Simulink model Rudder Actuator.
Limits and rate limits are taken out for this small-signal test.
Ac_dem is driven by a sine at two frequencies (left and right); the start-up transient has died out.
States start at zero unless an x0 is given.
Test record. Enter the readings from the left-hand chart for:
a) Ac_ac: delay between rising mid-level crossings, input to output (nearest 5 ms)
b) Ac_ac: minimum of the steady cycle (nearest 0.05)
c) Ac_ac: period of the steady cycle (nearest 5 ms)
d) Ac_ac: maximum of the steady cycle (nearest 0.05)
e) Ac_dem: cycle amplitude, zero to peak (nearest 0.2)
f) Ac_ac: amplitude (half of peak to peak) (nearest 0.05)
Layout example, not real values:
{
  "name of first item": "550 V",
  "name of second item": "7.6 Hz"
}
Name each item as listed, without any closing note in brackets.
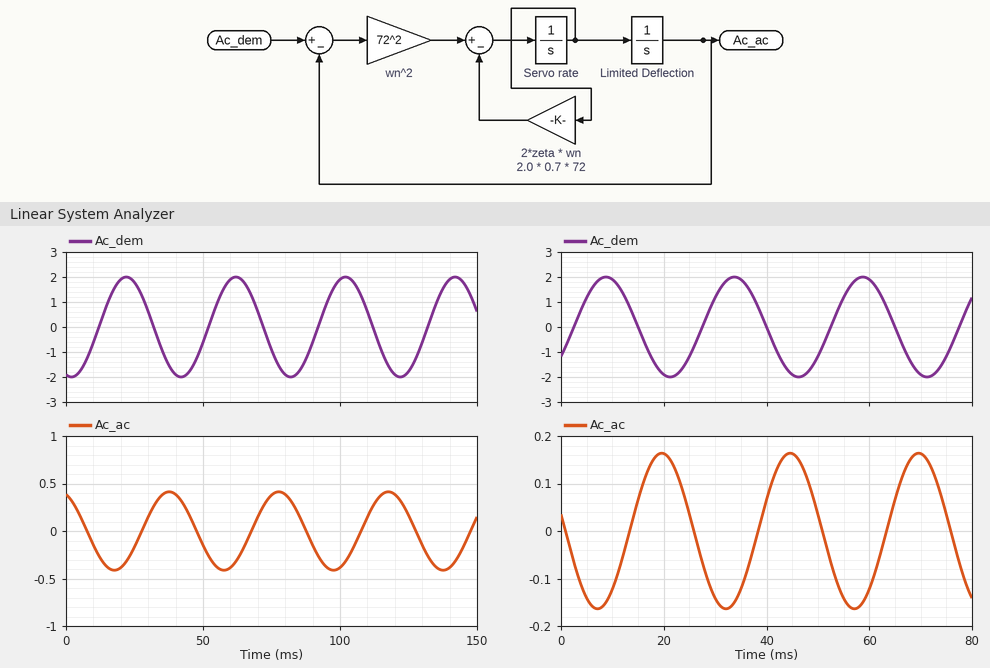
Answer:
{
  "Ac_ac: delay between rising mid-level crossings, input to output": "15 ms",
  "Ac_ac: minimum of the steady cycle": "-0.40",
  "Ac_ac: period of the steady cycle": "40 ms",
  "Ac_ac: maximum of the steady cycle": "0.40",
  "Ac_dem: cycle amplitude, zero to peak": "2.0",
  "Ac_ac: amplitude (half of peak to peak)": "0.40"
}
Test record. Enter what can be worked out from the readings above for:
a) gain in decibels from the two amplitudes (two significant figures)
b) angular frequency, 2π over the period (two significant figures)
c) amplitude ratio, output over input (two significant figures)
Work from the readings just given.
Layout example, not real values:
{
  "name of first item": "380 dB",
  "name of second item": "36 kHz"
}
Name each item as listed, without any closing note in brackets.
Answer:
{
  "gain in decibels from the two amplitudes": "-14 dB",
  "angular frequency, 2π over the period": "0.16 rad/ms",
  "amplitude ratio, output over input": "0.20"
}
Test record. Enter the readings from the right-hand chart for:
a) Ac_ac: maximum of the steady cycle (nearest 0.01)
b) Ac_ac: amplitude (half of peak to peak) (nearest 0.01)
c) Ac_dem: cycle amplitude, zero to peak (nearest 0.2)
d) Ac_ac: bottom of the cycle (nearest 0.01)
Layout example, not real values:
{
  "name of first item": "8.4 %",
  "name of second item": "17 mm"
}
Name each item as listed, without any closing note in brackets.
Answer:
{
  "Ac_ac: maximum of the steady cycle": "0.16",
  "Ac_ac: amplitude (half of peak to peak)": "0.16",
  "Ac_dem: cycle amplitude, zero to peak": "2.0",
  "Ac_ac: bottom of the cycle": "-0.16"
}
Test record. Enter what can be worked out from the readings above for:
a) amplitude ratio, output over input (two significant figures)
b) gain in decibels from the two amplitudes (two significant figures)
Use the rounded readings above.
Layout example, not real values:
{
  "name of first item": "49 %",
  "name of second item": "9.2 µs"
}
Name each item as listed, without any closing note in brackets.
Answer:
{
  "amplitude ratio, output over input": "0.080",
  "gain in decibels from the two amplitudes": "-22 dB"
}
